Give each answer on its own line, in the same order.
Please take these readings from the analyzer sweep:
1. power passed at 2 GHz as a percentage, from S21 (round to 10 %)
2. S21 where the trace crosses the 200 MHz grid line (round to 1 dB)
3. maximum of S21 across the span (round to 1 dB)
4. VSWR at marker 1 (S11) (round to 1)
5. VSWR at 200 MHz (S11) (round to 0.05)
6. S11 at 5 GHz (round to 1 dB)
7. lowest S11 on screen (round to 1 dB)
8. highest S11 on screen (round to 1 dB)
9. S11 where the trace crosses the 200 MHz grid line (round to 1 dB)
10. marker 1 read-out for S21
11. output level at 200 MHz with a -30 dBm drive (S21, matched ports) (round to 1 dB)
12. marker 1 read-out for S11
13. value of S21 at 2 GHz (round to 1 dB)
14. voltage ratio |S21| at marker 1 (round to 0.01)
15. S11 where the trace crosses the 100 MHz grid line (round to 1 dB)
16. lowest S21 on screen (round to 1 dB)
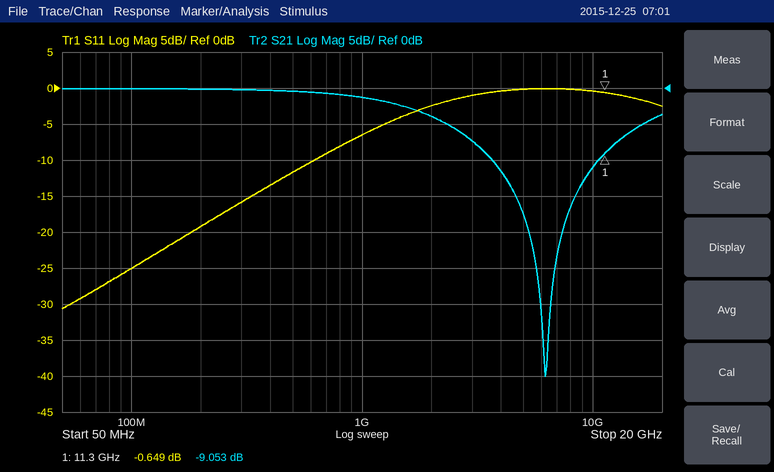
40 %
0 dB
0 dB
27
1.25
0 dB
-31 dB
0 dB
-19 dB
-9.053 dB
-30 dBm
-0.649 dB
-4 dB
0.35
-25 dB
-40 dB
